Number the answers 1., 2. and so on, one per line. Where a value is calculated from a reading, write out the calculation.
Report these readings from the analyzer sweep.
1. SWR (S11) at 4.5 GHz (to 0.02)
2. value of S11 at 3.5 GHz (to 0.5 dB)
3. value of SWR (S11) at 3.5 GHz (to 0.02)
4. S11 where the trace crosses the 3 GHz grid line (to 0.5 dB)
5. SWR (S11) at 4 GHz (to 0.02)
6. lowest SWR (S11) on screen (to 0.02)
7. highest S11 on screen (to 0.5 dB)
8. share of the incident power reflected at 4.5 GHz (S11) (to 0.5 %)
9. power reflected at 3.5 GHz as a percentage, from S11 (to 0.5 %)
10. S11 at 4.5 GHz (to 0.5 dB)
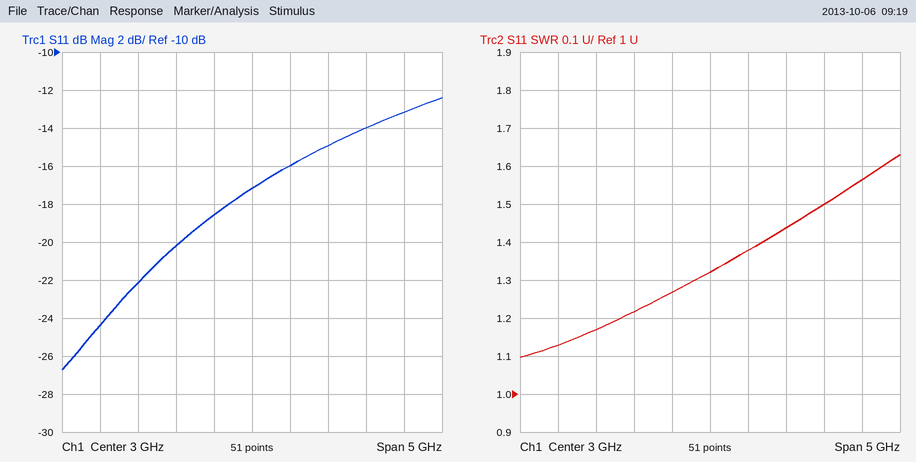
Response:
1. 1.50
2. -16.0 dB
3. 1.38
4. -17.0 dB
5. 1.44
6. 1.10
7. -12.5 dB
8. 10^(-14/10) ≈ 4.0 %
9. 10^(-16/10) ≈ 2.5 %
10. -14.0 dB
